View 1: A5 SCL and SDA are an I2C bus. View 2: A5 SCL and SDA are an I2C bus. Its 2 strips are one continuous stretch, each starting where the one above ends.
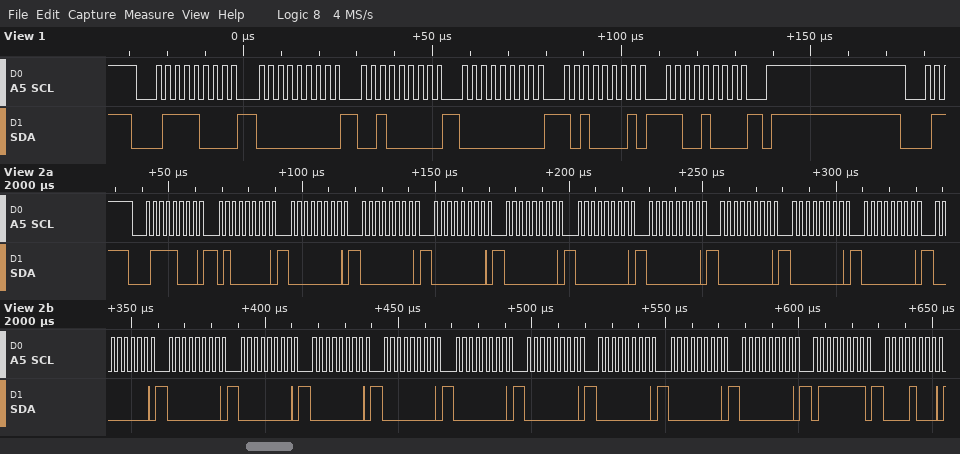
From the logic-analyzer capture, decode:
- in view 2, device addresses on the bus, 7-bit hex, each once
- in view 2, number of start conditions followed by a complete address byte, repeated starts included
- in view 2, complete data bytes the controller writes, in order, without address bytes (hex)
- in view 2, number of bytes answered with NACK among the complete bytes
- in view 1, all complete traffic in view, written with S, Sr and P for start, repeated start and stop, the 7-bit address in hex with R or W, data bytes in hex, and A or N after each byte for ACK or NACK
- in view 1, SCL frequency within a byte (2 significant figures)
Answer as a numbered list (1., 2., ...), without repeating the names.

1. 0x3C
2. 1
3. 40 00 00 00 00 00 00 00 00 00 00 00 00 00 00 00 00 00 00 00 7F 08
4. 0
5. S 3CW A 00 A 20 A 00 A A1 A C8 A P
6. 400 kHz
